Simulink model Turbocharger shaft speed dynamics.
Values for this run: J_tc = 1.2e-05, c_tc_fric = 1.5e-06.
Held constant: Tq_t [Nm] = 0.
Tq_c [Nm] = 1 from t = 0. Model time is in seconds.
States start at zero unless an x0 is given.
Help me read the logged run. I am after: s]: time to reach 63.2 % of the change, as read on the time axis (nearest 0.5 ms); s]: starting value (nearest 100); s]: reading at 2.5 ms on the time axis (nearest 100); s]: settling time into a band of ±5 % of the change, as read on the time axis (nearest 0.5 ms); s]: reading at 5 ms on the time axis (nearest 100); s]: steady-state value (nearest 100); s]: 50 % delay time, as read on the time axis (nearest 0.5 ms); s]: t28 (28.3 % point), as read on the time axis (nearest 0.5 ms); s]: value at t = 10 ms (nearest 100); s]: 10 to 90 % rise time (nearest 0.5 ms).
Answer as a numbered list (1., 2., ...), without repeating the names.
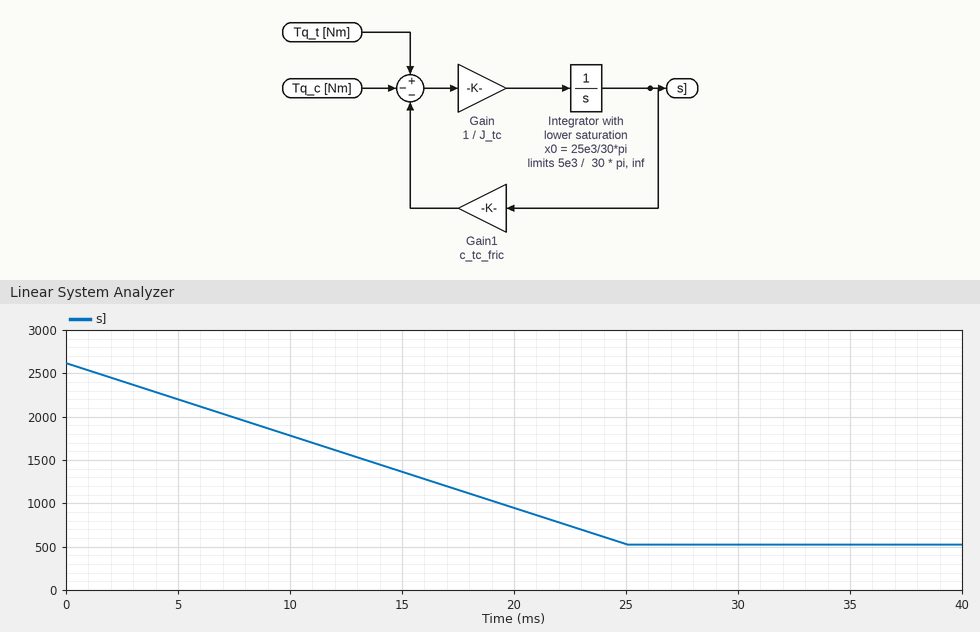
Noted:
1. 16.0 ms
2. 2600
3. 2400
4. 24.0 ms
5. 2200
6. 500
7. 12.5 ms
8. 7.0 ms
9. 1800
10. 20.0 ms
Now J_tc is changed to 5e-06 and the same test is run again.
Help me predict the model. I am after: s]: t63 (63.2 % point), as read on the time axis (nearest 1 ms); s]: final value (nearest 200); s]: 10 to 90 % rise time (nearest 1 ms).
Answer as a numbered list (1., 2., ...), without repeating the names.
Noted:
1. 7 ms
2. 600
3. 8 ms
